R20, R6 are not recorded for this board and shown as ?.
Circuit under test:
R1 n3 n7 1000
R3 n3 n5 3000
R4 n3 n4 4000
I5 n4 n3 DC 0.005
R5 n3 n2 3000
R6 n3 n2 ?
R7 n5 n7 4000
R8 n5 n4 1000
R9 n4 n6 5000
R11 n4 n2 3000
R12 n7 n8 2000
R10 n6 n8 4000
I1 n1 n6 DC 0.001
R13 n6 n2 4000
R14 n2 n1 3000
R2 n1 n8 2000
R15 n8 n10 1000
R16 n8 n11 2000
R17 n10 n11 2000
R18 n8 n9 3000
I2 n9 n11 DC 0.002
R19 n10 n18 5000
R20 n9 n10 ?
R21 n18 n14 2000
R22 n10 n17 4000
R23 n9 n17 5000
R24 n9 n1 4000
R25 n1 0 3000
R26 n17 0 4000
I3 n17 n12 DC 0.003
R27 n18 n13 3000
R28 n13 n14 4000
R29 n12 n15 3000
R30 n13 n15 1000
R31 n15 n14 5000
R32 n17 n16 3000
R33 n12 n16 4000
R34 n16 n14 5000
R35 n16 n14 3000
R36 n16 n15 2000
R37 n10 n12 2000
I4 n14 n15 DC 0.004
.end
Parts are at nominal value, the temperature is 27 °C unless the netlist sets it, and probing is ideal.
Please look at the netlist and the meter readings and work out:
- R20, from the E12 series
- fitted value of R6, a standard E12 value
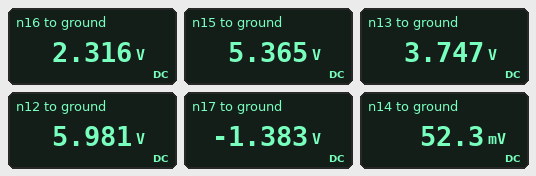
470 Ω
680 Ω
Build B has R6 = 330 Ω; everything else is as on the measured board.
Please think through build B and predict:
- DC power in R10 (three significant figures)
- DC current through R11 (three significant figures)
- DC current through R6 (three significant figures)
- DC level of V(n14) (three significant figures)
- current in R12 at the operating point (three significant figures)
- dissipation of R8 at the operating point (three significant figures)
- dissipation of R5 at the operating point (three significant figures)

97.8 µW
1.37 mA
1.81 mA
21.8 mV
199 µA
2.61 mW
119 µW
